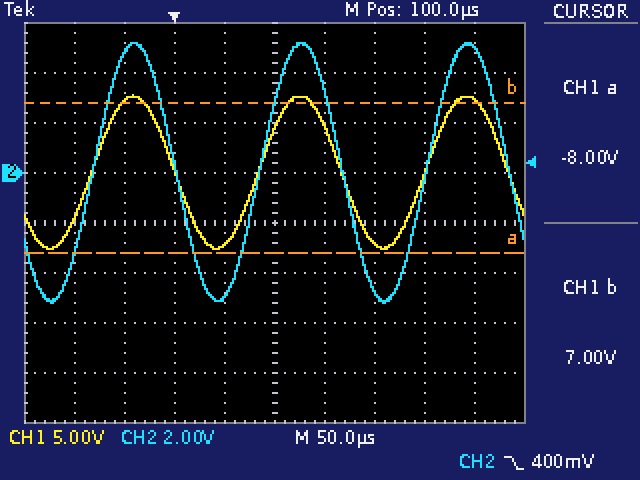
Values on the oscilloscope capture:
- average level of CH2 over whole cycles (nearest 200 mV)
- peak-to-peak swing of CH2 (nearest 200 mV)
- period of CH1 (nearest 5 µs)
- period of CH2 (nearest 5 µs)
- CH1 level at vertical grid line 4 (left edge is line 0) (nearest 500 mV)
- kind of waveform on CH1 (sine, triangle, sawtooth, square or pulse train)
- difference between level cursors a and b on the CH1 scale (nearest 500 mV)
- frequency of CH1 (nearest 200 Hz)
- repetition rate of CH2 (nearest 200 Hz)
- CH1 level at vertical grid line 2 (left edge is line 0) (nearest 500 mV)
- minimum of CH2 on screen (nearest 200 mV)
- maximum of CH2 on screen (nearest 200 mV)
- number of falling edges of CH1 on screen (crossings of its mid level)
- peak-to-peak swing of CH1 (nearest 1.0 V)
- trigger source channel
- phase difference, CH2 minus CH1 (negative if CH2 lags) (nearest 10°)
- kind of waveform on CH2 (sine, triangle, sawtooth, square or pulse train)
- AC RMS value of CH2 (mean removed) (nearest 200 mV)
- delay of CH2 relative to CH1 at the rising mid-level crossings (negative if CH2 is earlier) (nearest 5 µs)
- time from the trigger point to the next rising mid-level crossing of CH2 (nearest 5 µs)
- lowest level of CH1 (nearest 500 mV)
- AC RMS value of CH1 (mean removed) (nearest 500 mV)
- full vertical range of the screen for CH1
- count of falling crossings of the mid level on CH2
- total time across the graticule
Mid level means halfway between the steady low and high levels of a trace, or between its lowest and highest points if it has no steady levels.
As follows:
0.0 V
10.4 V
165 µs
165 µs
-7.0 V
sine
15.0 V
6.0 kHz
6.0 kHz
7.0 V
-5.2 V
5.2 V
3
15.0 V
CH2
0°
sine
3.6 V
0 µs
85 µs
-7.5 V
5.5 V
40 V
3
500 µs
